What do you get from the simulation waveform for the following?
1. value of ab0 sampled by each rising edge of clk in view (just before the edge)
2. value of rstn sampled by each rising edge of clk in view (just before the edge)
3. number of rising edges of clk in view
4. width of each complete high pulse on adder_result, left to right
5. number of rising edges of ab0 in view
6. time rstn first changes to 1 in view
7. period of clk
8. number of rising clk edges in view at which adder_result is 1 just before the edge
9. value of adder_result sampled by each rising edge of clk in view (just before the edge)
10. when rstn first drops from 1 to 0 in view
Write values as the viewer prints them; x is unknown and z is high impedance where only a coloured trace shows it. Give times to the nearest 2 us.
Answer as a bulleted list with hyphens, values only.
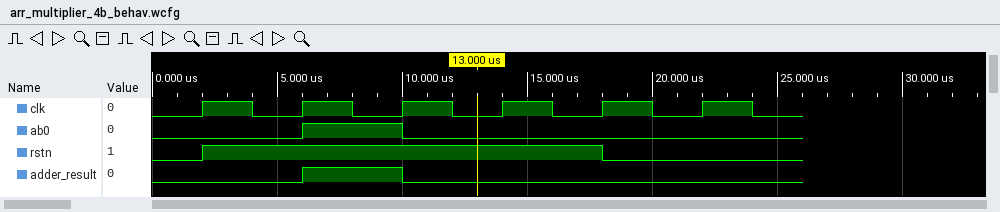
- 0 0 1 0 0 0
- 0 1 1 1 1 0
- 6
- 4 us
- 1
- 2 us
- 4 us
- 1
- 0 0 1 0 0 0
- 18 us
